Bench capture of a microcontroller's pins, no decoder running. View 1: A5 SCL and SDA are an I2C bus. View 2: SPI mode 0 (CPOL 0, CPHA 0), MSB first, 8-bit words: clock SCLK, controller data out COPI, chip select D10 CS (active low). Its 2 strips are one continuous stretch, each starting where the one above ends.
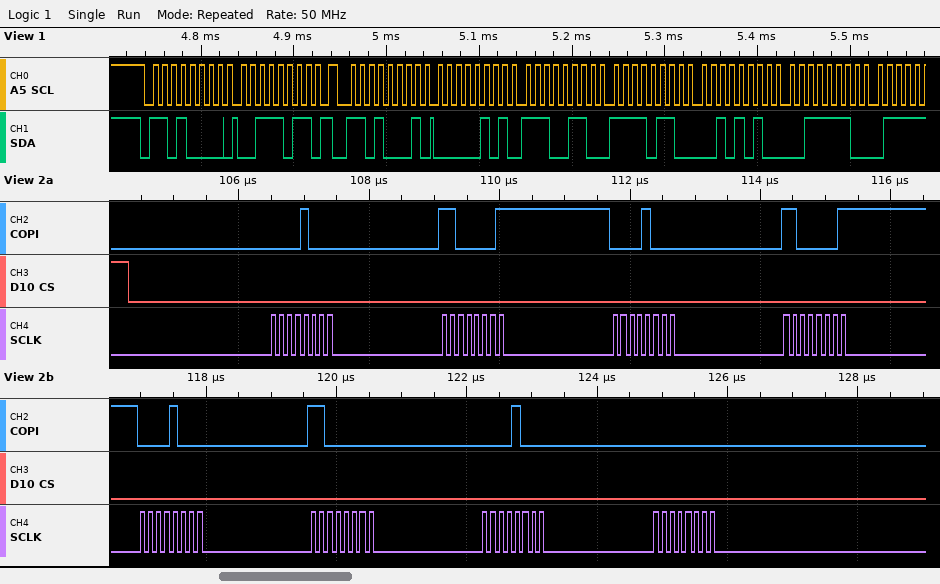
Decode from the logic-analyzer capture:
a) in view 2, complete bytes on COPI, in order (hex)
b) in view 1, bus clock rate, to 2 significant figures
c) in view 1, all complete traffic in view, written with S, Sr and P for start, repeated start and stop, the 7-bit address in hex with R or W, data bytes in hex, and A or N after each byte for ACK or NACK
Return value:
0x08 0xC1 0x08 0xC1 0x08 0xC0 0x08 0x00
100 kHz
S 68W A 3B A Sr 68R A 05 A E6 A F6 A 2A A 3E A
